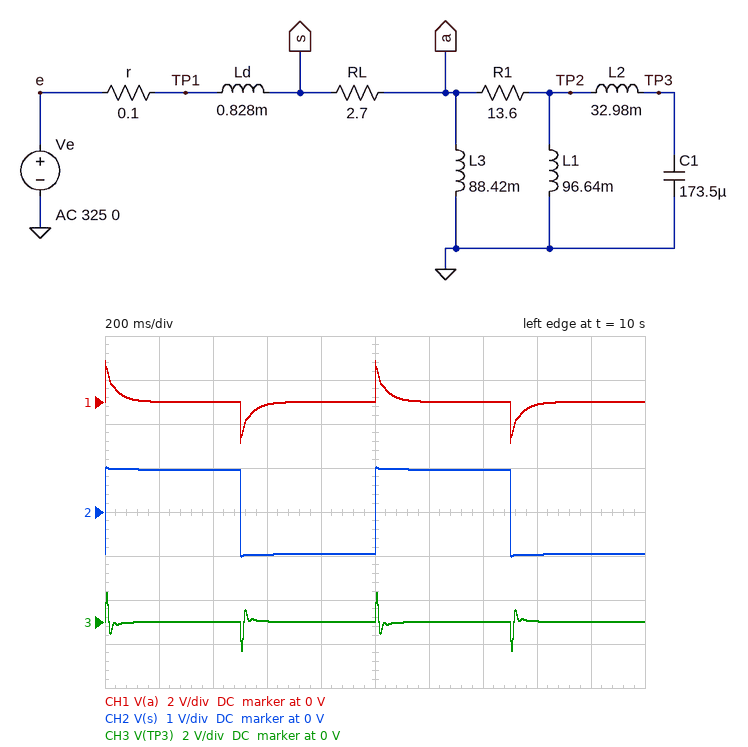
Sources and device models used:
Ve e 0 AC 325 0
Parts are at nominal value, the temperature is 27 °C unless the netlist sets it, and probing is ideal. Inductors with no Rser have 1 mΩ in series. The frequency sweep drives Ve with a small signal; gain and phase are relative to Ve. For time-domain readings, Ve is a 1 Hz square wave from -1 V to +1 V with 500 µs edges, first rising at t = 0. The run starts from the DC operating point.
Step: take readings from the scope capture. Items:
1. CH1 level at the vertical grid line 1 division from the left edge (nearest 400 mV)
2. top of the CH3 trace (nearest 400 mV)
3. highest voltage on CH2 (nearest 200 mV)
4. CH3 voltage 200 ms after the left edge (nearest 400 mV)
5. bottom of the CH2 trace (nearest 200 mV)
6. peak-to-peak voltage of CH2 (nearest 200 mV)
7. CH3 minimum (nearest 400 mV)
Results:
0 V
1.2 V
1.0 V
0 V
-1.0 V
2.0 V
-1.2 V
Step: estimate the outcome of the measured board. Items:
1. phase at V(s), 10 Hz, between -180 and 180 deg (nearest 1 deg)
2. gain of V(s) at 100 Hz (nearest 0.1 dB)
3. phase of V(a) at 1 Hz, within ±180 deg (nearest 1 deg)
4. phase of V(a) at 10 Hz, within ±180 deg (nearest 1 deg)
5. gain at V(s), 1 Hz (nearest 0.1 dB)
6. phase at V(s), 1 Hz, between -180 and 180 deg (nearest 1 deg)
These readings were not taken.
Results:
0 deg
-0.2 dB
76 deg
26 deg
-0.3 dB
0 deg
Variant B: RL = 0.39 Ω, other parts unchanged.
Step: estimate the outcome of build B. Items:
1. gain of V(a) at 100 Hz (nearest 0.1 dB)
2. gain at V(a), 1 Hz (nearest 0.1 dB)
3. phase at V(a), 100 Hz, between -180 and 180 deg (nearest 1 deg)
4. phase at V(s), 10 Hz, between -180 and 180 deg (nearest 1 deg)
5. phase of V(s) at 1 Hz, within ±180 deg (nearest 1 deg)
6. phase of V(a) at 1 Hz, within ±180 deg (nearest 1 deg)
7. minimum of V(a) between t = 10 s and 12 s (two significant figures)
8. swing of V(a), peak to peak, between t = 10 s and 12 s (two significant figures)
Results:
-0.4 dB
-2.7 dB
0 deg
1 deg
6 deg
40 deg
-1.8 V
3.6 V
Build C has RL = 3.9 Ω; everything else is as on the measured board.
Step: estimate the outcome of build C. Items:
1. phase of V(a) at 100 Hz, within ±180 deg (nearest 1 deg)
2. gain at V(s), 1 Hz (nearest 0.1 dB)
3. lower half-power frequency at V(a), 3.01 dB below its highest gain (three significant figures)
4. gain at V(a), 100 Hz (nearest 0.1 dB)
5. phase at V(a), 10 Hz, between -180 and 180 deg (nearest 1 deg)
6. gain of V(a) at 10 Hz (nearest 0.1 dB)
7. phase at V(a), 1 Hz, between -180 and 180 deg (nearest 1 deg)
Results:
9 deg
-0.2 dB
11.3 Hz
-1.8 dB
34 deg
-3.5 dB
80 deg
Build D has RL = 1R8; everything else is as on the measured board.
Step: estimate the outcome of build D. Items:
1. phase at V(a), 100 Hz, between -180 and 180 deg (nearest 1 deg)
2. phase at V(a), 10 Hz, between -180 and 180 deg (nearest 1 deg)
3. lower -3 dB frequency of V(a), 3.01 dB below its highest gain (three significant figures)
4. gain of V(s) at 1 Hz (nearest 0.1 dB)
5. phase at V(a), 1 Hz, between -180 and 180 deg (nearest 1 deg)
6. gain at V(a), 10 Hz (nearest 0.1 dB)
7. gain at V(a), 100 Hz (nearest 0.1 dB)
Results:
4 deg
19 deg
4.09 Hz
-0.4 dB
71 deg
-1.5 dB
-1.0 dB
